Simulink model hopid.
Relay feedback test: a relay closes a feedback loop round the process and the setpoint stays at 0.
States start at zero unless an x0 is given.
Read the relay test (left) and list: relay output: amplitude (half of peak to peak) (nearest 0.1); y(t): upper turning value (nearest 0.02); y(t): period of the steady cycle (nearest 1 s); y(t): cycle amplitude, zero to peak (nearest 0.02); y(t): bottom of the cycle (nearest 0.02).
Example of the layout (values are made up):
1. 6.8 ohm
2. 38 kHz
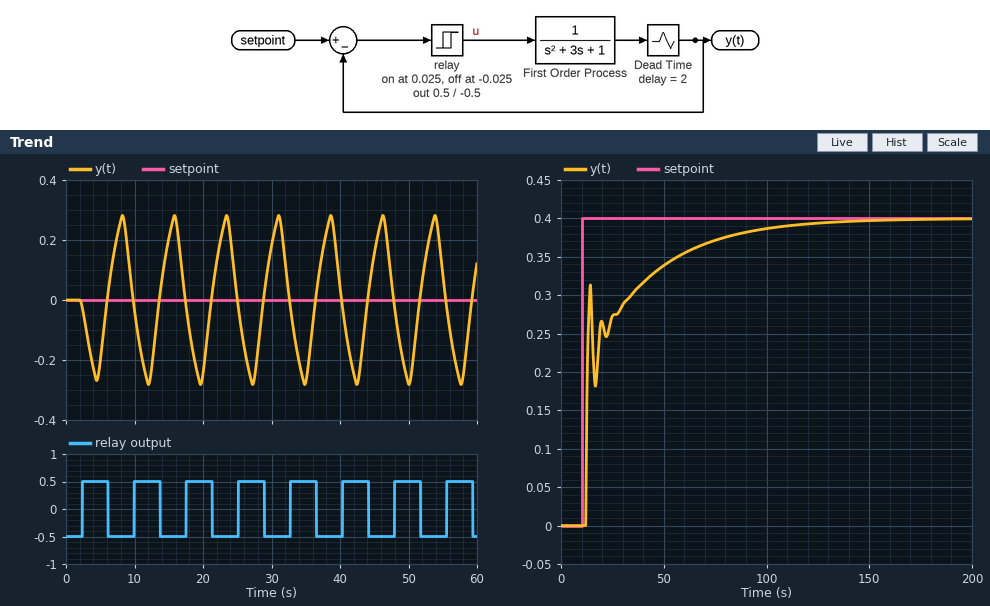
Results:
1. 0.5
2. 0.28
3. 8 s
4. 0.28
5. -0.28
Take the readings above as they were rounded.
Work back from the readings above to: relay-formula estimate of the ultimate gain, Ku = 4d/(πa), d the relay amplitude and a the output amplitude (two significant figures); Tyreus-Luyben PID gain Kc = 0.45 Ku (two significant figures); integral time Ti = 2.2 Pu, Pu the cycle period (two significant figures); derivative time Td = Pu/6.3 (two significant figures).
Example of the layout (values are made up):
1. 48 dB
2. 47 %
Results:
1. 2.3
2. 1.0
3. 18 s
4. 1.3 s
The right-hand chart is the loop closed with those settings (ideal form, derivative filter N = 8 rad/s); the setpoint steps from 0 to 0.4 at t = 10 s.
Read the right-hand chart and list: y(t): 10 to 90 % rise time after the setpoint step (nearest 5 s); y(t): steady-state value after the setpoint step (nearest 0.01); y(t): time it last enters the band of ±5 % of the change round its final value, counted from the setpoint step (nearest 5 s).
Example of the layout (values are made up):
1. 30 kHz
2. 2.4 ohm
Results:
1. 50 s
2. 0.40
3. 75 s
